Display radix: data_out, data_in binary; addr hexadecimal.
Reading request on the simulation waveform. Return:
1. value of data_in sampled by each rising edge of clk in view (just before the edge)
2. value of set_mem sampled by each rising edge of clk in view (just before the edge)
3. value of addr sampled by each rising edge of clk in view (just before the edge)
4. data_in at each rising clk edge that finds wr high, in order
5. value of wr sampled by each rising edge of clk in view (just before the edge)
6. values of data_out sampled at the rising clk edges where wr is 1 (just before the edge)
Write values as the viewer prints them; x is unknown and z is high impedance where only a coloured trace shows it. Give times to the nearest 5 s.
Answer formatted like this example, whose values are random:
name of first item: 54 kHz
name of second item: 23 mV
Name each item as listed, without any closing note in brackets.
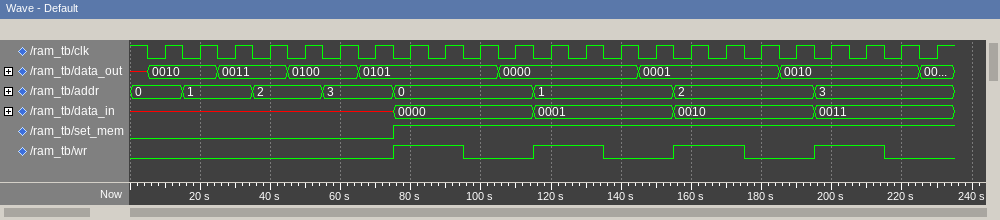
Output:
value of data_in sampled by each rising edge of clk in view: x, x, x, x, x, x, x, 0000, 0000, 0000, 0000, 0001, 0001, 0001, 0001, 0010, 0010, 0010, 0010, 0011, 0011, 0011, 0011
value of set_mem sampled by each rising edge of clk in view: 0 0 0 0 0 0 0 1 1 1 1 1 1 1 1 1 1 1 1 1 1 1 1
value of addr sampled by each rising edge of clk in view: 0, 1, 1, 2, 2, 3, 3, 0, 0, 0, 0, 1, 1, 1, 1, 2, 2, 2, 2, 3, 3, 3, 3
data_in at each rising clk edge that finds wr high, in order: 0000, 0000, 0001, 0001, 0010, 0010, 0011, 0011
value of wr sampled by each rising edge of clk in view: 0 0 0 0 0 0 0 1 1 0 0 1 1 0 0 1 1 0 0 1 1 0 0
values of data_out sampled at the rising clk edges where wr is 1: 0101, 0101, 0000, 0000, 0001, 0001, 0010, 0010
